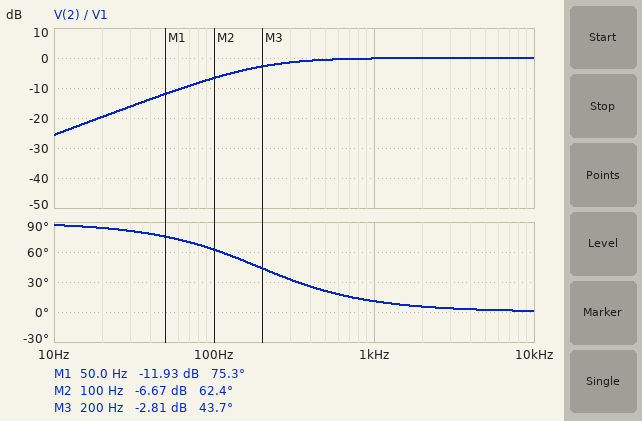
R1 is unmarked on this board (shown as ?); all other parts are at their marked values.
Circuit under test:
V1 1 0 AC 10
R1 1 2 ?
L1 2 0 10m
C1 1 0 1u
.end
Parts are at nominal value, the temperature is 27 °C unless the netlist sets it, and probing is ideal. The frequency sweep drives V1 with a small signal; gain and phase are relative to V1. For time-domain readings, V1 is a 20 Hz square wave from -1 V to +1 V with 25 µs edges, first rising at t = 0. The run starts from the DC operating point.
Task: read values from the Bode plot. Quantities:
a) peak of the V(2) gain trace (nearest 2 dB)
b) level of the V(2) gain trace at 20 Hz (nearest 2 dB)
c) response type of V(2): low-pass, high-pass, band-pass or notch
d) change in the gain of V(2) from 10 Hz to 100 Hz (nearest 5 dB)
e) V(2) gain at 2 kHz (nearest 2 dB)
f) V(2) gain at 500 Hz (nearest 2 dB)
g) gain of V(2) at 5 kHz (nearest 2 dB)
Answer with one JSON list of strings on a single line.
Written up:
["0 dB", "-20 dB", "high-pass", "20 dB", "0 dB", "0 dB", "0 dB"]
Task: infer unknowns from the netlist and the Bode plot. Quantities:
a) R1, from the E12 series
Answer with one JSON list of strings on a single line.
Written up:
["12 Ω"]
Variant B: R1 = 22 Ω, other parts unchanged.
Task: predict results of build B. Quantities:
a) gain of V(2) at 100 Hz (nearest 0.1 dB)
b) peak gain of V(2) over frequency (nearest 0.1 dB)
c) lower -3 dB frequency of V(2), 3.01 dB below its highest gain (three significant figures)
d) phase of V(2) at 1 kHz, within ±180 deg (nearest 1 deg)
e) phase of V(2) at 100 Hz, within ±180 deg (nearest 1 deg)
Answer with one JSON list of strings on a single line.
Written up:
["-11.2 dB", "0 dB", "350 Hz", "19 deg", "74 deg"]
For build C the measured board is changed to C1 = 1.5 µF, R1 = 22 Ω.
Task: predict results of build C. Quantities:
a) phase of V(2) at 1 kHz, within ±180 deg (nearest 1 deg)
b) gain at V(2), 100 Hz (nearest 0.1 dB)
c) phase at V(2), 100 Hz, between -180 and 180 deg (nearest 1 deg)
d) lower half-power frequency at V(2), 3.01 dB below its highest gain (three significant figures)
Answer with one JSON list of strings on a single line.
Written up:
["19 deg", "-11.2 dB", "74 deg", "350 Hz"]
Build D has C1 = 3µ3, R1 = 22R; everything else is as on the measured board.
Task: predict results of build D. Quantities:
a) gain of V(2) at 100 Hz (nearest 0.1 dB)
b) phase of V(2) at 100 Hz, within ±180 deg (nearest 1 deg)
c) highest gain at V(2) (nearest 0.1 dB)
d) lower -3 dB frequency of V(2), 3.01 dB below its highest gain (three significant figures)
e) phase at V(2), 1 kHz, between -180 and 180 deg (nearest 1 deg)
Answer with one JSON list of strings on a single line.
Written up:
["-11.2 dB", "74 deg", "0 dB", "350 Hz", "19 deg"]
